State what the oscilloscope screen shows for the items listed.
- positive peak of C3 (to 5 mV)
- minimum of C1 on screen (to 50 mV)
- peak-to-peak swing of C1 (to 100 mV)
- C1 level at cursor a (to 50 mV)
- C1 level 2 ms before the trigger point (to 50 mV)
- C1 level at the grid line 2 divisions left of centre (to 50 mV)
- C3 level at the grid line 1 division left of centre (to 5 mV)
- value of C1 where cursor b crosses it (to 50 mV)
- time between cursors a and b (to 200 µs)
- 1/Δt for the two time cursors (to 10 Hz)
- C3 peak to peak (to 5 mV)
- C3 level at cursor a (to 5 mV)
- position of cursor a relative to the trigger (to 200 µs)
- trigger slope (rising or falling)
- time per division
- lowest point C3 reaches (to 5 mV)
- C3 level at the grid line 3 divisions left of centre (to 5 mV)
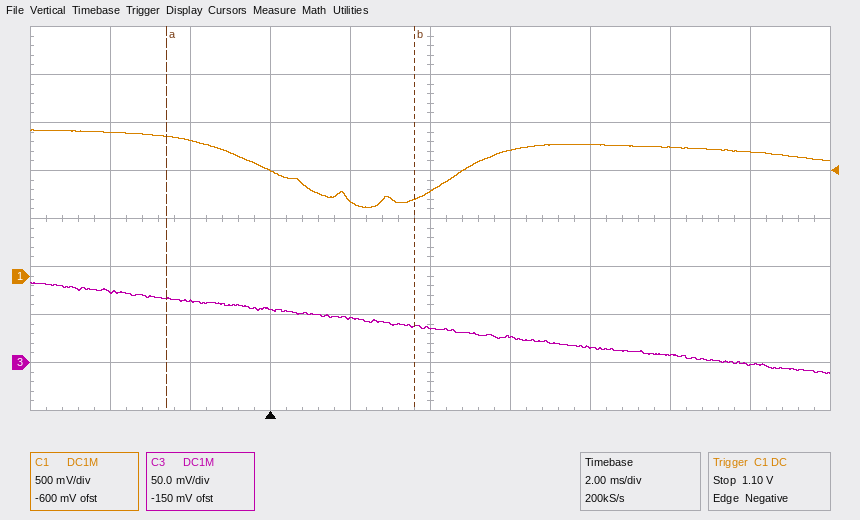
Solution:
85 mV
700 mV
800 mV
1.45 V
1.40 V
1.10 V
45 mV
800 mV
6.2 ms
160 Hz
95 mV
65 mV
-2.6 ms
falling
2 ms
-10 mV
65 mV
